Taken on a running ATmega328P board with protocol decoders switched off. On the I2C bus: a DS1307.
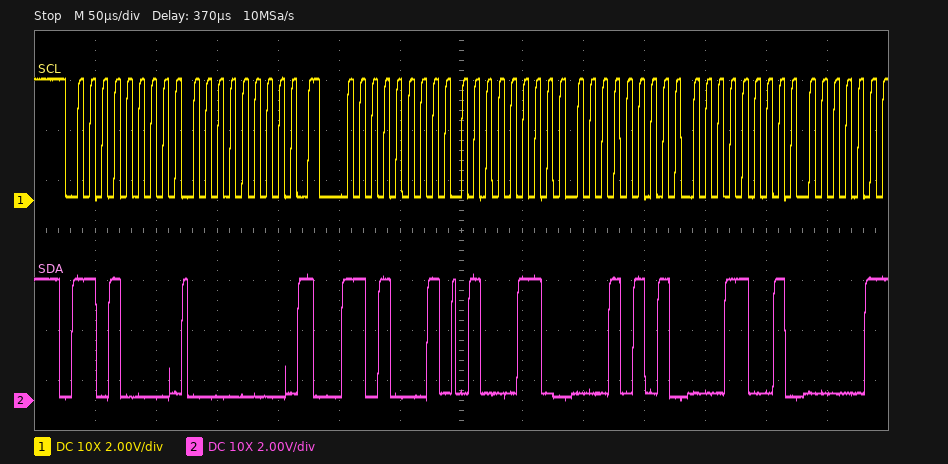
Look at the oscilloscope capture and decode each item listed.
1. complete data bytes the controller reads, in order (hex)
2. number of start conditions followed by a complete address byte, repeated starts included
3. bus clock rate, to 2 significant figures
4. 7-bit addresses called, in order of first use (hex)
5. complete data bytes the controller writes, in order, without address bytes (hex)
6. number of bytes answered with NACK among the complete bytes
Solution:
46 15 19
2
100 kHz
0x68
00
0
